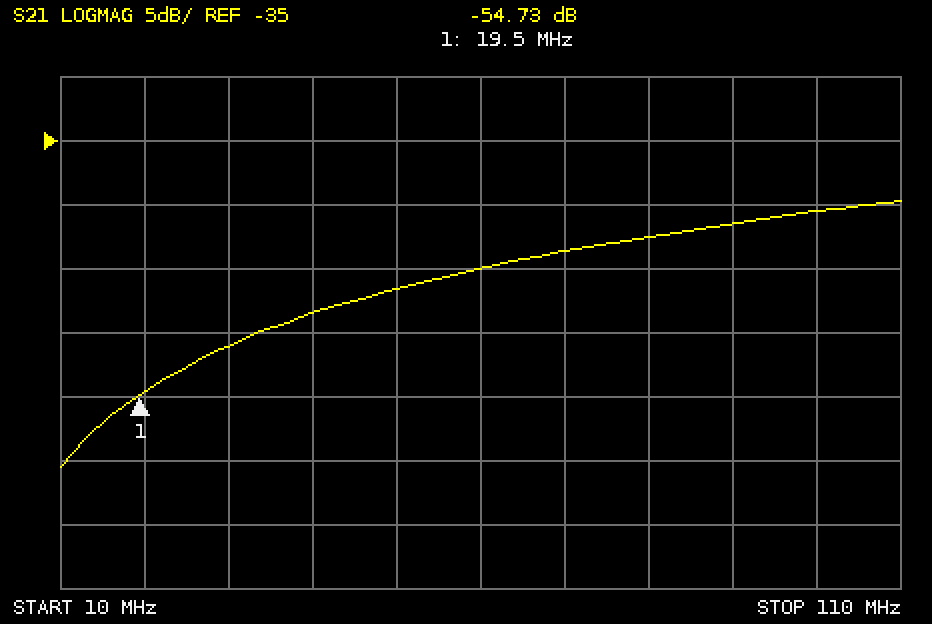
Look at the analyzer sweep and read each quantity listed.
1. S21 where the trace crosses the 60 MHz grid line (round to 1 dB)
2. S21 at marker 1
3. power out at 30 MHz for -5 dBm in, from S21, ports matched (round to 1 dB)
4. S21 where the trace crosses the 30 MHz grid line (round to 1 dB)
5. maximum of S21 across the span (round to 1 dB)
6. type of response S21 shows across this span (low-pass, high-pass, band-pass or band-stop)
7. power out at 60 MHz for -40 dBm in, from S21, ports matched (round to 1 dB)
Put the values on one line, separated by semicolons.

-45 dB; -54.73 dB; -56 dBm; -51 dB; -40 dB; high-pass; -85 dBm
